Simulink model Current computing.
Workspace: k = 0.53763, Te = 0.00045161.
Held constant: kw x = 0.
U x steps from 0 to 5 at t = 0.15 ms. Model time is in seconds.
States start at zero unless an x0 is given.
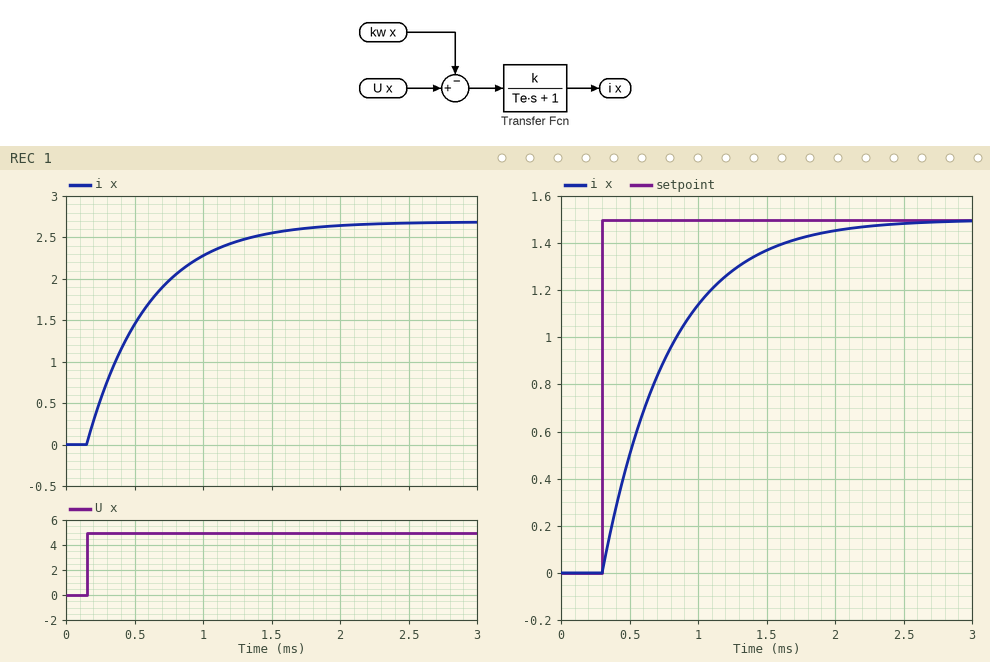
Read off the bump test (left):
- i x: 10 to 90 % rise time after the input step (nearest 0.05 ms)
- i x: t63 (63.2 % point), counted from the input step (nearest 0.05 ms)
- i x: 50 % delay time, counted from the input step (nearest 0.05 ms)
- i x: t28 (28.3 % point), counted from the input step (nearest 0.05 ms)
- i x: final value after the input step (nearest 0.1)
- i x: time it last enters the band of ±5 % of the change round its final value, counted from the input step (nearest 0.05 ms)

1.00 ms
0.45 ms
0.30 ms
0.15 ms
2.7
1.35 ms
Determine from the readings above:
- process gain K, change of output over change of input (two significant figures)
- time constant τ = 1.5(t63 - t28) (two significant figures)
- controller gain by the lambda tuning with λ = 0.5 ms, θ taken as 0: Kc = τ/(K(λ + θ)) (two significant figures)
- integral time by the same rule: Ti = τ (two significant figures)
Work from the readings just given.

0.54
0.45 ms
1.7
0.45 ms
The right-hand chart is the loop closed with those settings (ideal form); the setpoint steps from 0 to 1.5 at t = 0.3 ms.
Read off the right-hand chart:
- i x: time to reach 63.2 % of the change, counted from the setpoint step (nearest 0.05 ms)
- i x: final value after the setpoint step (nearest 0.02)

0.50 ms
1.50
